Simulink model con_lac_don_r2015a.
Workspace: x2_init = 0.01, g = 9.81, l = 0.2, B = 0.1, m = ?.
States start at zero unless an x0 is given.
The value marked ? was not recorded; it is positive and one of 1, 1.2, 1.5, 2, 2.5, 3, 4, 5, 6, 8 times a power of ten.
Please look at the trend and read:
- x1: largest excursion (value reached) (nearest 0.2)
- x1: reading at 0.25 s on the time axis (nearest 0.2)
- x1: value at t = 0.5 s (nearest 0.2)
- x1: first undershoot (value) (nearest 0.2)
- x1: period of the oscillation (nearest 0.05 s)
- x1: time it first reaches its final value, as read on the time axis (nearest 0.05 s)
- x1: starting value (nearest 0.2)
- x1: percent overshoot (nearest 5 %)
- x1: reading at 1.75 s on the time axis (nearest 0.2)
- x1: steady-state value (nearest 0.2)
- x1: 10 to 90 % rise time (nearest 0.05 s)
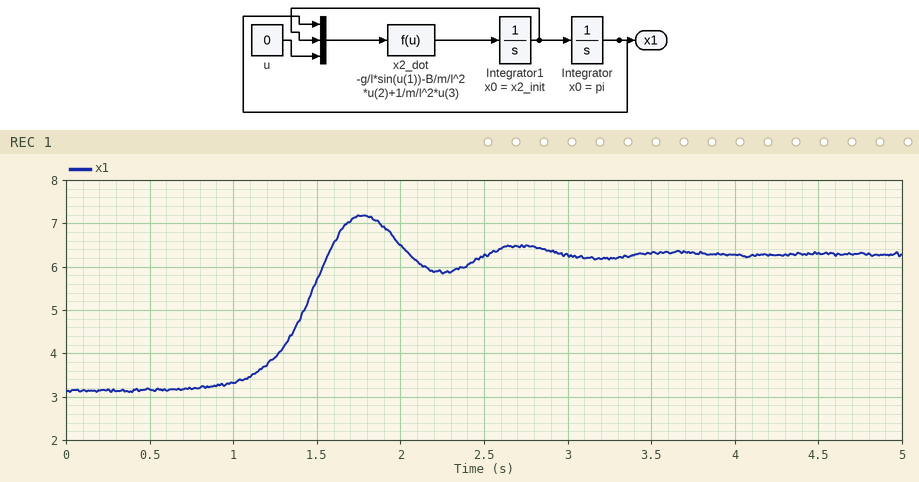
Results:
7.2
3.2
3.2
5.8
0.95 s
1.55 s
3.2
30 %
7.2
6.2
0.45 s
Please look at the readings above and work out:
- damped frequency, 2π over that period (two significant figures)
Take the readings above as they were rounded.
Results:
6.6 rad/s
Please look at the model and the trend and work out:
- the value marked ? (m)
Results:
0.8
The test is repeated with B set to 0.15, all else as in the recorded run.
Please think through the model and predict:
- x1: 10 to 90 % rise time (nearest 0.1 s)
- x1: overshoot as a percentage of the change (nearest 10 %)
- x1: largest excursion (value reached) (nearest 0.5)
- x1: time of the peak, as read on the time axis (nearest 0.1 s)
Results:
0.5 s
20 %
7.0
2.0 s
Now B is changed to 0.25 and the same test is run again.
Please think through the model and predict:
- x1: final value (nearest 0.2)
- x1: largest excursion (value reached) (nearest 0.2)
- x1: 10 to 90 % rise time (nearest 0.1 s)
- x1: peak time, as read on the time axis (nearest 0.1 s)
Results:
6.2
6.4
0.7 s
2.4 s
